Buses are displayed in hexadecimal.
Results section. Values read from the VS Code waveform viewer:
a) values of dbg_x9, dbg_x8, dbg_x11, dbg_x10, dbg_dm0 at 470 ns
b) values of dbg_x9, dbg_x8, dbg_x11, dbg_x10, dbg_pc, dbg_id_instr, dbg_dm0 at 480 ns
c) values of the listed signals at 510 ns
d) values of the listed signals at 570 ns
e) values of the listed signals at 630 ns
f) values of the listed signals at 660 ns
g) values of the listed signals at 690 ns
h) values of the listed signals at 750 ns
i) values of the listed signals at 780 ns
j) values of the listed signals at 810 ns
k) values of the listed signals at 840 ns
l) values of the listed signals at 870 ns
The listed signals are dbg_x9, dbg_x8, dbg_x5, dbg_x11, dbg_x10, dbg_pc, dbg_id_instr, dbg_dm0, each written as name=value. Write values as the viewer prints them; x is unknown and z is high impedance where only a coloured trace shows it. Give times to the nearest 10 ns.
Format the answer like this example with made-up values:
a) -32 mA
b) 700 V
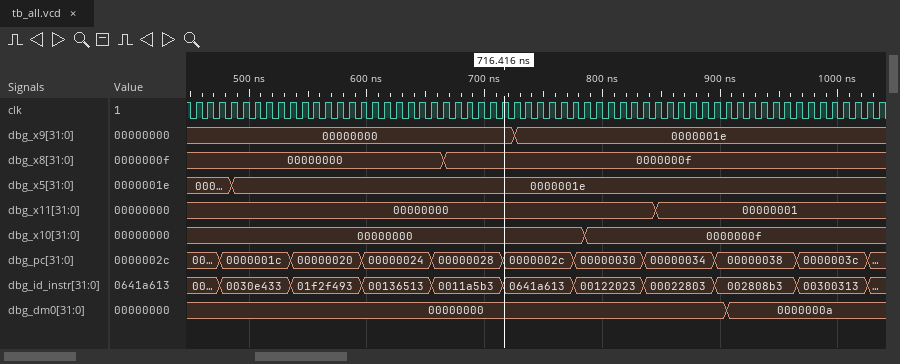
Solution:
a) dbg_x9=00000000, dbg_x8=00000000, dbg_x11=00000000, dbg_x10=00000000, dbg_dm0=00000000
b) dbg_x9=00000000, dbg_x8=00000000, dbg_x11=00000000, dbg_x10=00000000, dbg_pc=0000001c, dbg_id_instr=0030e433, dbg_dm0=00000000
c) dbg_x9=00000000, dbg_x8=00000000, dbg_x5=0000001e, dbg_x11=00000000, dbg_x10=00000000, dbg_pc=0000001c, dbg_id_instr=0030e433, dbg_dm0=00000000
d) dbg_x9=00000000, dbg_x8=00000000, dbg_x5=0000001e, dbg_x11=00000000, dbg_x10=00000000, dbg_pc=00000020, dbg_id_instr=01f2f493, dbg_dm0=00000000
e) dbg_x9=00000000, dbg_x8=00000000, dbg_x5=0000001e, dbg_x11=00000000, dbg_x10=00000000, dbg_pc=00000024, dbg_id_instr=00136513, dbg_dm0=00000000
f) dbg_x9=00000000, dbg_x8=00000000, dbg_x5=0000001e, dbg_x11=00000000, dbg_x10=00000000, dbg_pc=00000028, dbg_id_instr=0011a5b3, dbg_dm0=00000000
g) dbg_x9=00000000, dbg_x8=0000000f, dbg_x5=0000001e, dbg_x11=00000000, dbg_x10=00000000, dbg_pc=00000028, dbg_id_instr=0011a5b3, dbg_dm0=00000000
h) dbg_x9=0000001e, dbg_x8=0000000f, dbg_x5=0000001e, dbg_x11=00000000, dbg_x10=00000000, dbg_pc=0000002c, dbg_id_instr=0641a613, dbg_dm0=00000000
i) dbg_x9=0000001e, dbg_x8=0000000f, dbg_x5=0000001e, dbg_x11=00000000, dbg_x10=00000000, dbg_pc=00000030, dbg_id_instr=00122023, dbg_dm0=00000000
j) dbg_x9=0000001e, dbg_x8=0000000f, dbg_x5=0000001e, dbg_x11=00000000, dbg_x10=0000000f, dbg_pc=00000030, dbg_id_instr=00122023, dbg_dm0=00000000
k) dbg_x9=0000001e, dbg_x8=0000000f, dbg_x5=0000001e, dbg_x11=00000000, dbg_x10=0000000f, dbg_pc=00000034, dbg_id_instr=00022803, dbg_dm0=00000000
l) dbg_x9=0000001e, dbg_x8=0000000f, dbg_x5=0000001e, dbg_x11=00000001, dbg_x10=0000000f, dbg_pc=00000034, dbg_id_instr=00022803, dbg_dm0=00000000
